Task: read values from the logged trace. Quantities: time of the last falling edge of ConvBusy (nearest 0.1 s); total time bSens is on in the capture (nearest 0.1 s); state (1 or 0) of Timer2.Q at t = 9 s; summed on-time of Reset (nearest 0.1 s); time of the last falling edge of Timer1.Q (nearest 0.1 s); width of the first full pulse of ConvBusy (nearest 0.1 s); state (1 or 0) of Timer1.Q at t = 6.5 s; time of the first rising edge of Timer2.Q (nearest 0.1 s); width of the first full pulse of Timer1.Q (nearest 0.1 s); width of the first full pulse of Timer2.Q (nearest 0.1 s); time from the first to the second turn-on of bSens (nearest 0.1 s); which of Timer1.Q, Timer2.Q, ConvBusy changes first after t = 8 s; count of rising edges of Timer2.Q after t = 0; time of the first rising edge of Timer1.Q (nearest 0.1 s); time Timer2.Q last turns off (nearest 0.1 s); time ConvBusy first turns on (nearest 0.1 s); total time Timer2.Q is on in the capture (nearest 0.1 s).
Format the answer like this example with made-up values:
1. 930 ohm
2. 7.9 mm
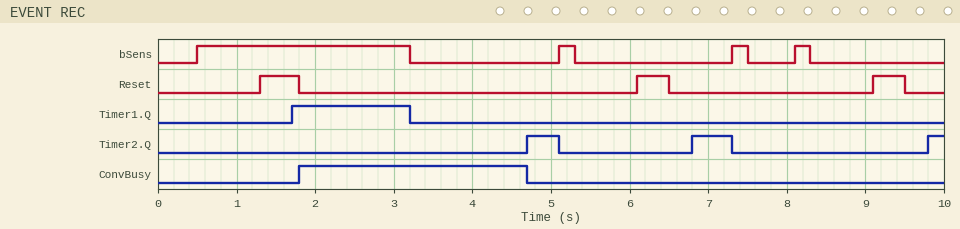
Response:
1. 4.7 s
2. 3.3 s
3. 0
4. 1.3 s
5. 3.2 s
6. 2.9 s
7. 0
8. 4.7 s
9. 1.5 s
10. 0.4 s
11. 4.6 s
12. Timer2.Q
13. 3
14. 1.7 s
15. 7.3 s
16. 1.8 s
17. 1.1 s
